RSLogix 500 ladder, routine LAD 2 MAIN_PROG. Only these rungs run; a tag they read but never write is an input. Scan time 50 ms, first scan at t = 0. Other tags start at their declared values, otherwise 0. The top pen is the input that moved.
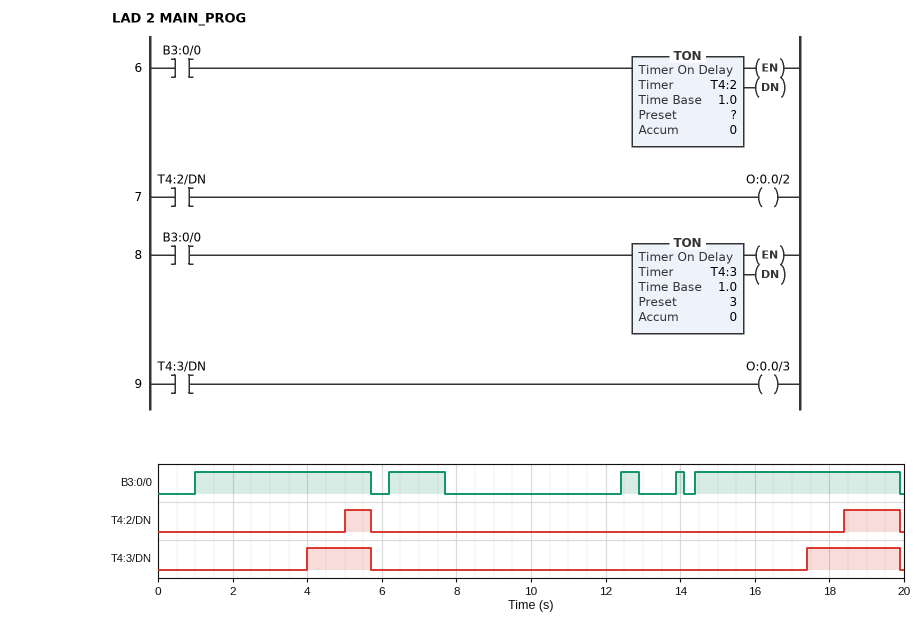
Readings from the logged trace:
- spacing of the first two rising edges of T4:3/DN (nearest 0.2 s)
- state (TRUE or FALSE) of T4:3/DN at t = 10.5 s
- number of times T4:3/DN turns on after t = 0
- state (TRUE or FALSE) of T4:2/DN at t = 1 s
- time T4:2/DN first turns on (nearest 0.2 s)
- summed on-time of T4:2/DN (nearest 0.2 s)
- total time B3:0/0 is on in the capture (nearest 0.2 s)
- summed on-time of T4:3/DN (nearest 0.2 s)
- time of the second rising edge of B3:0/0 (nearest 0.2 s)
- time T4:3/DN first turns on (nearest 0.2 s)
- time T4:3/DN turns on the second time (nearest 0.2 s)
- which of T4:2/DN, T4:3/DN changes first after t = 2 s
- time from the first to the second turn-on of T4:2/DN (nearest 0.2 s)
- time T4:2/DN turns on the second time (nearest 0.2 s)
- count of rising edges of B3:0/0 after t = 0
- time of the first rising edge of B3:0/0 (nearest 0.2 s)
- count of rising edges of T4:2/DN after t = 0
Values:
13.4 s
FALSE
2
FALSE
5.0 s
2.2 s
12.4 s
4.2 s
6.2 s
4.0 s
17.4 s
T4:3/DN
13.4 s
18.4 s
5
1.0 s
2
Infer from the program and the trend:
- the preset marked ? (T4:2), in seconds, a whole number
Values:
4 s
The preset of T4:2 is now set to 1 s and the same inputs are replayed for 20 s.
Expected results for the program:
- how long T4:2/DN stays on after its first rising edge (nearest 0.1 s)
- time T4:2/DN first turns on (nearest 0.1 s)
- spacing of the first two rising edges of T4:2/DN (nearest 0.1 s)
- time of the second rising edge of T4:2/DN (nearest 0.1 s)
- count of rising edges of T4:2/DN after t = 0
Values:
3.7 s
2.0 s
5.2 s
7.2 s
3
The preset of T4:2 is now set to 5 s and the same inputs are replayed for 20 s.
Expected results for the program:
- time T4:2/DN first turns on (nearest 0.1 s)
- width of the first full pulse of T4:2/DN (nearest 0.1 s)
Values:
19.4 s
0.5 s
